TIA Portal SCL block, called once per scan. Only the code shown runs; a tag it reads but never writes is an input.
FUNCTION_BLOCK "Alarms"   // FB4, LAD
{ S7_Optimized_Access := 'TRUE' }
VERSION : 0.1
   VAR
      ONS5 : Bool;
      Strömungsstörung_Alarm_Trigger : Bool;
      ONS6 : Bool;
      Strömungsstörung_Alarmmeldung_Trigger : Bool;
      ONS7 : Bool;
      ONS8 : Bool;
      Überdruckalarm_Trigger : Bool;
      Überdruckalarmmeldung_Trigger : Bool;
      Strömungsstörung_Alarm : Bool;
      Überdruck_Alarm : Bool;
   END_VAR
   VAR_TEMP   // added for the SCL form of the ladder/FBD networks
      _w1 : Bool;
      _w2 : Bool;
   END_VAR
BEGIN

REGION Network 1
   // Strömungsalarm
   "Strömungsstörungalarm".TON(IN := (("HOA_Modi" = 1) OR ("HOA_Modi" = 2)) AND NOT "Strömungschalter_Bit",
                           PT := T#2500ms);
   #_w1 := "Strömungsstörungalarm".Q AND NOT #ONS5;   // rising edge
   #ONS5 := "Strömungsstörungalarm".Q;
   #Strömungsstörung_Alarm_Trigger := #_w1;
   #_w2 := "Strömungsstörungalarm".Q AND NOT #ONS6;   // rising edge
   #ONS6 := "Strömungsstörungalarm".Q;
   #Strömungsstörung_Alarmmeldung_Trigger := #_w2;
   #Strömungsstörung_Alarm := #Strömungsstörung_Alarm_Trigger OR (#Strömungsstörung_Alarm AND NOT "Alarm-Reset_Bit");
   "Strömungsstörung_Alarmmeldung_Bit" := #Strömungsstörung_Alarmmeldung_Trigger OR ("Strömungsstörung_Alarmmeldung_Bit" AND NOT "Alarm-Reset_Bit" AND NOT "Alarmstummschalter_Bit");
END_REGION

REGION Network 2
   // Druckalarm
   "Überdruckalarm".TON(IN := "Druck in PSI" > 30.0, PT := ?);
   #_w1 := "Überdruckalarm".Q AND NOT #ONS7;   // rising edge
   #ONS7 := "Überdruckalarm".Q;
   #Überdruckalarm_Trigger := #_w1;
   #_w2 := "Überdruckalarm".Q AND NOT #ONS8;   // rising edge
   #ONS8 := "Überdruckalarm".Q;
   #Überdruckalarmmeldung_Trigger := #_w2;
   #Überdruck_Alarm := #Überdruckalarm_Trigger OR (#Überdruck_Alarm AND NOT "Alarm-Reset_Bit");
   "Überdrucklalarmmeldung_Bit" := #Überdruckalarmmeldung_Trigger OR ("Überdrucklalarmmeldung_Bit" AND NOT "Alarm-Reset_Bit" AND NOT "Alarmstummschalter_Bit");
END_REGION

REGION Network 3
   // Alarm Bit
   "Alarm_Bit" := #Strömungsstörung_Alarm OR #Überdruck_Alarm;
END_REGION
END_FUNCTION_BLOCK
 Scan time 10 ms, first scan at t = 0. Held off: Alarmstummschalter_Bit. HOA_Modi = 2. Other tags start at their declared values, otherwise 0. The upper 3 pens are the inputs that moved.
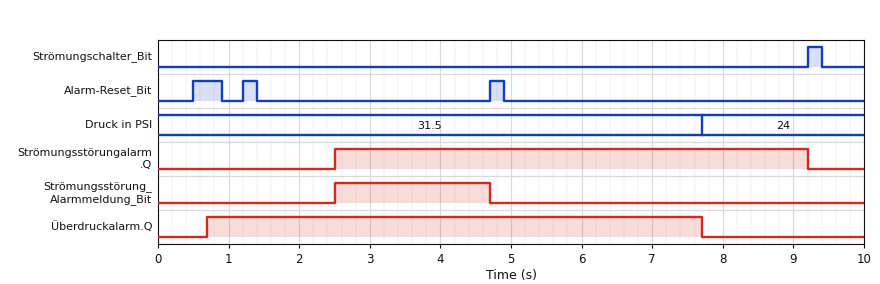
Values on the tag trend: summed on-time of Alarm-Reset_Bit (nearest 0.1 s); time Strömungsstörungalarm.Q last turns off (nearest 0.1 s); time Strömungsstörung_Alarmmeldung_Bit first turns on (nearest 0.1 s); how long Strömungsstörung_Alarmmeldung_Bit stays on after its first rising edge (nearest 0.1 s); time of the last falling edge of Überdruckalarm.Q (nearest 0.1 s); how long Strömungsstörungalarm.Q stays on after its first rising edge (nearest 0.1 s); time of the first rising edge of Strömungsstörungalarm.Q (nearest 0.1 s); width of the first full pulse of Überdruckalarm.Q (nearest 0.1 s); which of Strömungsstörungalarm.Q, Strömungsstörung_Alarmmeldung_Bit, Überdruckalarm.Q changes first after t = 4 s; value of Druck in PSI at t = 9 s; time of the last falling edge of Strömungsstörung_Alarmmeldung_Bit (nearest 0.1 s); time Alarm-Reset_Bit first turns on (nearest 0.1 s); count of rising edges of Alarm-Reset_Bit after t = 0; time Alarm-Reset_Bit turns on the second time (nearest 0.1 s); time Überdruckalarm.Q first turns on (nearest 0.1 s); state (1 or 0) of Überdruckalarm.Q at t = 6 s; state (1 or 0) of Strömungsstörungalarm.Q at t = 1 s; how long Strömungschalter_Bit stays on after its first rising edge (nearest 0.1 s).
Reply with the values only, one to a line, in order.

0.8 s
9.2 s
2.5 s
2.2 s
7.7 s
6.7 s
2.5 s
7.0 s
Strömungsstörung_Alarmmeldung_Bit
24
4.7 s
0.5 s
3
1.2 s
0.7 s
1
0
0.2 s
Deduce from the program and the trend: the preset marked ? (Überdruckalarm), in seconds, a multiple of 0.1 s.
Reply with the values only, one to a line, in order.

0.7 s
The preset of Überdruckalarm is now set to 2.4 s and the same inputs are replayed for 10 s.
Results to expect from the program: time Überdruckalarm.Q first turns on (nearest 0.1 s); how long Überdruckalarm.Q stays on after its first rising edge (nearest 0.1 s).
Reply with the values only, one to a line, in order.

2.4 s
5.3 s
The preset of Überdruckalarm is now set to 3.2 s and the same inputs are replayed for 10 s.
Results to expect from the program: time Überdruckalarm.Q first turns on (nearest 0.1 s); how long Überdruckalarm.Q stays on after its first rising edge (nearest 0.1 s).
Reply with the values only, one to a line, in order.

3.2 s
4.5 s
